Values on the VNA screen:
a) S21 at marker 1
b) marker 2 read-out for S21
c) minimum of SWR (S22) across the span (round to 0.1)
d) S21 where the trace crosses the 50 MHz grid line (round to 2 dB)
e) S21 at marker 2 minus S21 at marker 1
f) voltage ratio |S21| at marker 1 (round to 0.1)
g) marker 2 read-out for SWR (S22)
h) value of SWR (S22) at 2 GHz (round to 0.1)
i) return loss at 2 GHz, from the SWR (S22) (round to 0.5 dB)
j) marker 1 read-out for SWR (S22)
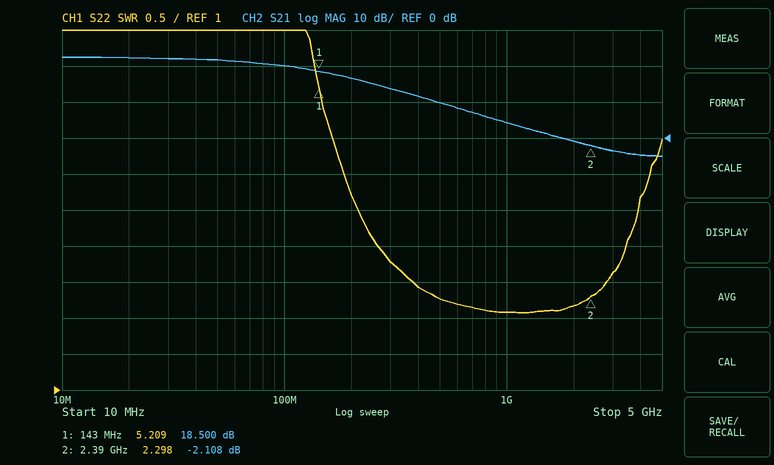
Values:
18.500 dB
-2.108 dB
2.1
22 dB
-20.608 dB
8.4
2.298
2.2
8.5 dB
5.209
